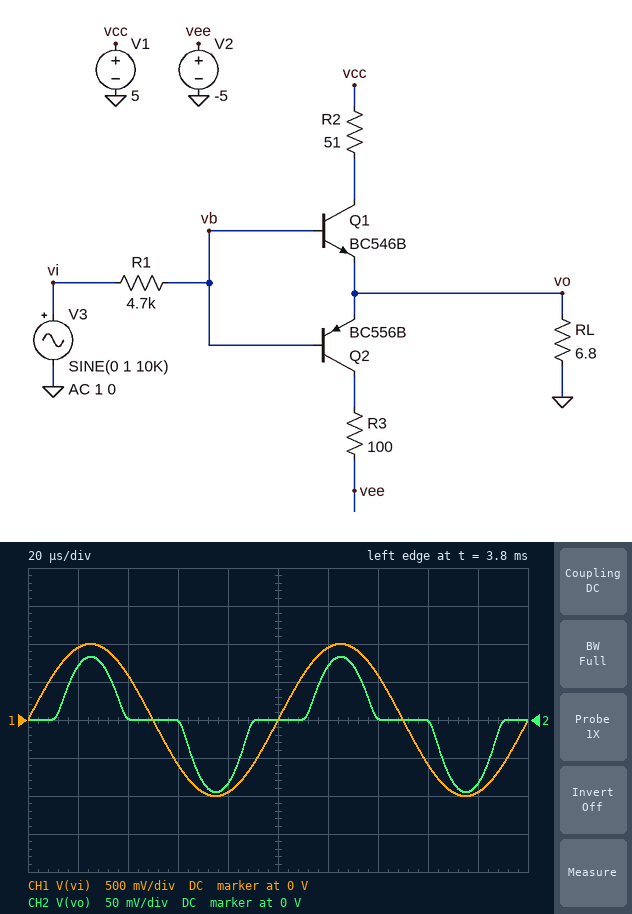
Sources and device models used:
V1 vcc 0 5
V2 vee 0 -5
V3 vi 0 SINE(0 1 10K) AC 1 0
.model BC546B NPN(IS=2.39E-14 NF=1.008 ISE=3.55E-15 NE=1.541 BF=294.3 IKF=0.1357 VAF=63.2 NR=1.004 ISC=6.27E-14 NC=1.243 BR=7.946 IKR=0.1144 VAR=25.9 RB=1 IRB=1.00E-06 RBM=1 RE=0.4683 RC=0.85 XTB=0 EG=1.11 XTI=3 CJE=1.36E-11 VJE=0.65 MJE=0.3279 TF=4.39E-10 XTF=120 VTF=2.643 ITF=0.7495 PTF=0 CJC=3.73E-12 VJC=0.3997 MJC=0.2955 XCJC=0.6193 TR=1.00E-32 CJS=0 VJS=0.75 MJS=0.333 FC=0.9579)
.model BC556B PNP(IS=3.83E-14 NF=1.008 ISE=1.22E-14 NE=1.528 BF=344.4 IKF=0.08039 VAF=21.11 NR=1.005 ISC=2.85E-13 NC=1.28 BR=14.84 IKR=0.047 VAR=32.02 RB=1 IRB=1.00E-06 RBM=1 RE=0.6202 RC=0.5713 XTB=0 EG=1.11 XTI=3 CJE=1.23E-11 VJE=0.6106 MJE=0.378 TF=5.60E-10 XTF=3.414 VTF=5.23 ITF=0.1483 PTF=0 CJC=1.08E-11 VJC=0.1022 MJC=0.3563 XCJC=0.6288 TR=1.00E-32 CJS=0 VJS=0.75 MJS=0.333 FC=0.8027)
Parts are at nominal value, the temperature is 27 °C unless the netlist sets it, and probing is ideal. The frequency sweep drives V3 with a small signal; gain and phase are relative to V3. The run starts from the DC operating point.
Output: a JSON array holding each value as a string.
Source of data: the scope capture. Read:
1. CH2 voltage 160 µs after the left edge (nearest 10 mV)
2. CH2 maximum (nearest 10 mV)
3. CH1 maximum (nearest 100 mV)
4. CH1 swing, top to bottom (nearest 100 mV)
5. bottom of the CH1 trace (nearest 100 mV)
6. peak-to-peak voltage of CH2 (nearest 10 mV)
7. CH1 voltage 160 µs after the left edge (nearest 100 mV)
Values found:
["0 V", "80 mV", "1.0 V", "2.0 V", "-1.0 V", "180 mV", "-600 mV"]
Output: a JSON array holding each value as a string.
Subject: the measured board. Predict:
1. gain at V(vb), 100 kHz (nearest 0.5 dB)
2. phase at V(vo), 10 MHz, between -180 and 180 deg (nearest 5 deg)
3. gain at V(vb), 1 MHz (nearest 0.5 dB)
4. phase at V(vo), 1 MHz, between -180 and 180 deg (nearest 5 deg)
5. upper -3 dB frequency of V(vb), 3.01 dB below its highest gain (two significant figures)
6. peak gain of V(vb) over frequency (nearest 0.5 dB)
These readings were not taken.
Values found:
["0 dB", "5 deg", "-2.5 dB", "50 deg", "1.1 MHz", "0 dB"]
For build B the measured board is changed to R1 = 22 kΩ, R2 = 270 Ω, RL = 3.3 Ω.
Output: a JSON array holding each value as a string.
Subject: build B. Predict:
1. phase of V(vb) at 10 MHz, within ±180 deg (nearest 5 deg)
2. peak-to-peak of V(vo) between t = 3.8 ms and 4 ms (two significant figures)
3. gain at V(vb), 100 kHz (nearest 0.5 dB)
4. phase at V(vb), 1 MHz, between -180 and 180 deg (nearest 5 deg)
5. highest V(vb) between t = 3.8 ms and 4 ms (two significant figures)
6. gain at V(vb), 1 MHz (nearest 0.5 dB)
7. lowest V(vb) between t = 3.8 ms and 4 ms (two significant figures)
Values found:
["-90 deg", "31 mV", "-0.5 dB", "-75 deg", "690 mV", "-12.5 dB", "-690 mV"]
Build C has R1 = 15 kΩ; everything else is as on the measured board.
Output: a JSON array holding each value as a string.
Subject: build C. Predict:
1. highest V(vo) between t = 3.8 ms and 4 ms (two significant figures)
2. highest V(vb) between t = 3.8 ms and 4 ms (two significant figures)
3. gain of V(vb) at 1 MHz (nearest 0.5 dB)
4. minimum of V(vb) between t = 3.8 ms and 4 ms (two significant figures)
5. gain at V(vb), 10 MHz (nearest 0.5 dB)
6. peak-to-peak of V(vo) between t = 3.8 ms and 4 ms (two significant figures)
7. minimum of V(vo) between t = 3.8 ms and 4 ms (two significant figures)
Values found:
["37 mV", "720 mV", "-9.5 dB", "-720 mV", "-29.0 dB", "83 mV", "-46 mV"]
